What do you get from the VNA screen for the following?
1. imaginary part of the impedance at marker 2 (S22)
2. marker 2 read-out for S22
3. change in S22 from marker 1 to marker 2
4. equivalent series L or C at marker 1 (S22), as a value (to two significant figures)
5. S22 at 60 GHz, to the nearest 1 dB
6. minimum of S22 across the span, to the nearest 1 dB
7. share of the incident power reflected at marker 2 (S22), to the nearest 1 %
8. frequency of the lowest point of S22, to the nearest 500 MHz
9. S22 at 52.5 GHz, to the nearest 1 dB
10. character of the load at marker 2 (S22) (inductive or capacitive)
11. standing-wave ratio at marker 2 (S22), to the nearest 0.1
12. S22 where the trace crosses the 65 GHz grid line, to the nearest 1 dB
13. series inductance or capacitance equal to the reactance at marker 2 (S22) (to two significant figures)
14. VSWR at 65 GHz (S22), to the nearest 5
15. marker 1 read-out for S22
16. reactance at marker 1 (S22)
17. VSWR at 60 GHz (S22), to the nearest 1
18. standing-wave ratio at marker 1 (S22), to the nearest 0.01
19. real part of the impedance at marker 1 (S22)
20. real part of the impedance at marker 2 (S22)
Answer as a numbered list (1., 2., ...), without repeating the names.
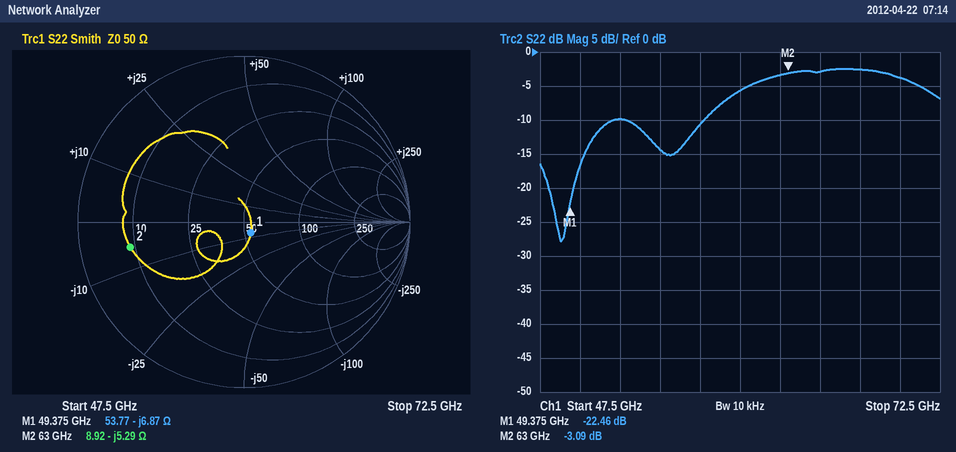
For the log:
1. -5.29 Ω
2. -3.09 dB
3. 19.37 dB
4. 470 fF
5. -6 dB
6. -28 dB
7. 49 %
8. 49.0 GHz
9. -10 dB
10. capacitive
11. 5.7
12. -3 dB
13. 480 fF
14. 5
15. -22.46 dB
16. -6.87 Ω
17. 3
18. 1.16
19. 53.77 Ω
20. 8.92 Ω
